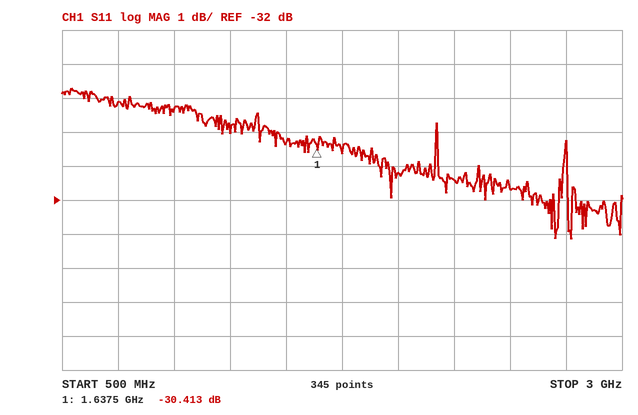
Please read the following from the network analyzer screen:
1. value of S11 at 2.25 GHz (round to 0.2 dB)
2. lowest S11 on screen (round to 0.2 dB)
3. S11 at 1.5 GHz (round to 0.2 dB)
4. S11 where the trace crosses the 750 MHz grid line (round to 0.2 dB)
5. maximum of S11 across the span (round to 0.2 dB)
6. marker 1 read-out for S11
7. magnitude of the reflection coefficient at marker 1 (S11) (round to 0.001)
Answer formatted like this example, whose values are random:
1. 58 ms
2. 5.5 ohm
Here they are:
1. -31.4 dB
2. -33.2 dB
3. -30.4 dB
4. -29.2 dB
5. -28.8 dB
6. -30.413 dB
7. 0.030
